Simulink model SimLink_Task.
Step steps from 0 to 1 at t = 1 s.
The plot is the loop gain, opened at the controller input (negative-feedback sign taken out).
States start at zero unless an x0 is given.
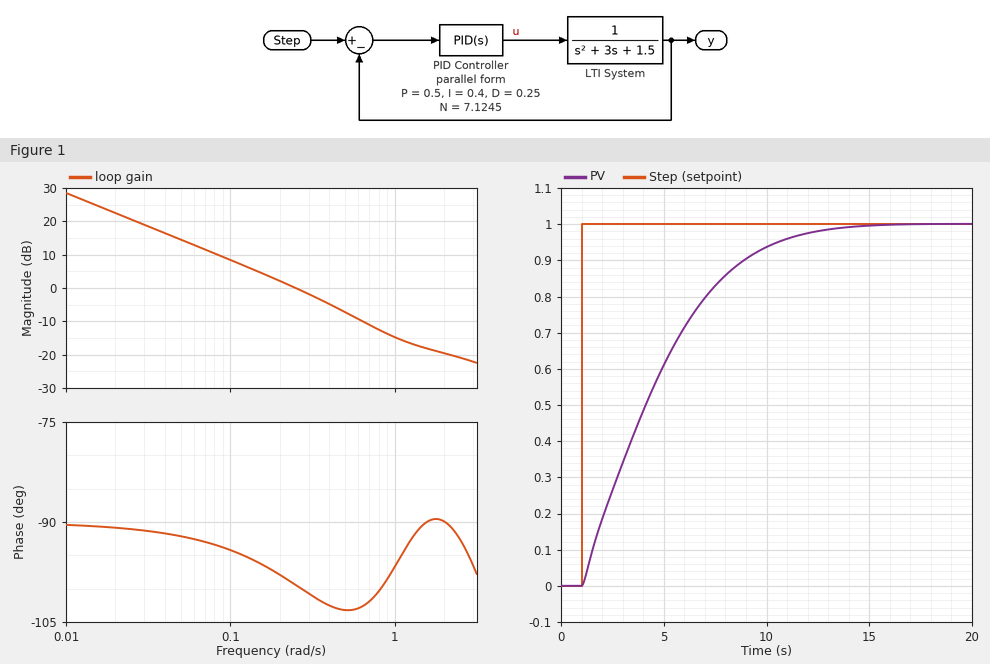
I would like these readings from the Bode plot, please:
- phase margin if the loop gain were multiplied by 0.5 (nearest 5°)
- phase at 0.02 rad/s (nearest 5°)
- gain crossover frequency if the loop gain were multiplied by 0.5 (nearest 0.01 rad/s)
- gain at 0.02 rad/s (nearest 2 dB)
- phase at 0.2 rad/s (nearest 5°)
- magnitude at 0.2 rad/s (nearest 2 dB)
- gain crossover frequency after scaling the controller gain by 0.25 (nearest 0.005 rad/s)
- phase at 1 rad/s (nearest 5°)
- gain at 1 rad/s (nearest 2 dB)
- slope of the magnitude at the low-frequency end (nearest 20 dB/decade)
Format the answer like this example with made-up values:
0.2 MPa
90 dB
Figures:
85°
-90°
0.13 rad/s
22 dB
-100°
2 dB
0.065 rad/s
-95°
-14 dB
-20 dB/decade
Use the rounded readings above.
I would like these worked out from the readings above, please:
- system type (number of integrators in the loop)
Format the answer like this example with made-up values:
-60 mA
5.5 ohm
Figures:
1
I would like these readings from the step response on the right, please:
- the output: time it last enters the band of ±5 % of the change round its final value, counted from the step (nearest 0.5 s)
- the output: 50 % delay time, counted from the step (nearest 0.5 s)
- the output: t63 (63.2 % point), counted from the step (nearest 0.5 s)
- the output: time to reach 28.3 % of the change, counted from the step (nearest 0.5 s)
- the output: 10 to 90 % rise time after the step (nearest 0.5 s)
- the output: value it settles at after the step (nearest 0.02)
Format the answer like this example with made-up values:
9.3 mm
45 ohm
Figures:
9.5 s
3.0 s
4.0 s
1.5 s
7.5 s
1.00
